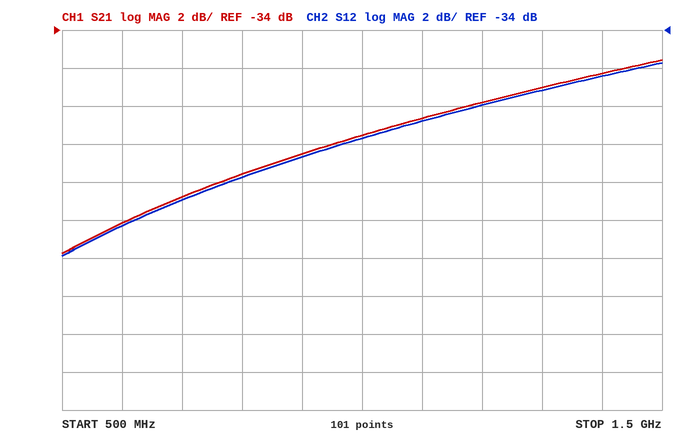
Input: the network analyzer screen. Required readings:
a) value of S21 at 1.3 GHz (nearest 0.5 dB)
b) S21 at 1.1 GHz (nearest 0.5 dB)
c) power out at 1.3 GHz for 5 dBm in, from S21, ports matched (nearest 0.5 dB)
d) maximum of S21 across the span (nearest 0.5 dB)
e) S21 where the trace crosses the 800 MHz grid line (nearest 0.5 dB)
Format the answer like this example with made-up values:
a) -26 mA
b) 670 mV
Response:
a) -37.0 dB
b) -38.5 dB
c) -32.0 dBm
d) -35.5 dB
e) -41.5 dB
